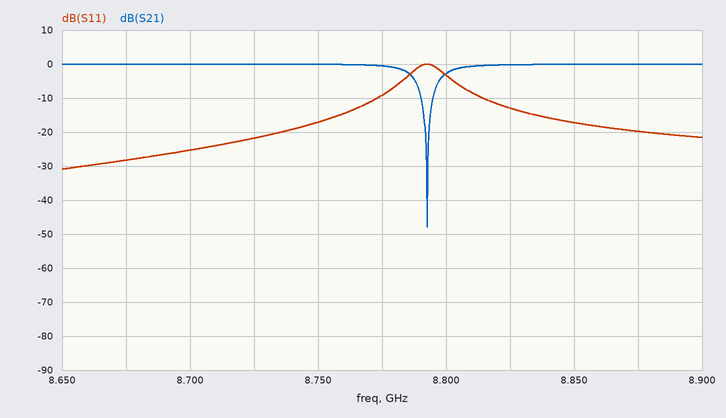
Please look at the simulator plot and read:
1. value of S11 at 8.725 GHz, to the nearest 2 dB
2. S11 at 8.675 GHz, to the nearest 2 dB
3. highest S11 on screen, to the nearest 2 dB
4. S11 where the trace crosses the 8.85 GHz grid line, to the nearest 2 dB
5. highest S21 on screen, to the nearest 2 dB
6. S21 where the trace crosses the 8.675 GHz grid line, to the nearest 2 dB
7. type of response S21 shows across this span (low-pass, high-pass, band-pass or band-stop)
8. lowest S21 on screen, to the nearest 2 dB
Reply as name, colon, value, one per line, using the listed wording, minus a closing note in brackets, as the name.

value of S11 at 8.725 GHz, to the nearest 2 dB: -22 dB
S11 at 8.675 GHz, to the nearest 2 dB: -28 dB
highest S11 on screen, to the nearest 2 dB: 0 dB
S11 where the trace crosses the 8.85 GHz grid line, to the nearest 2 dB: -18 dB
highest S21 on screen, to the nearest 2 dB: 0 dB
S21 where the trace crosses the 8.675 GHz grid line, to the nearest 2 dB: 0 dB
type of response S21 shows across this span: band-stop
lowest S21 on screen, to the nearest 2 dB: -48 dB
